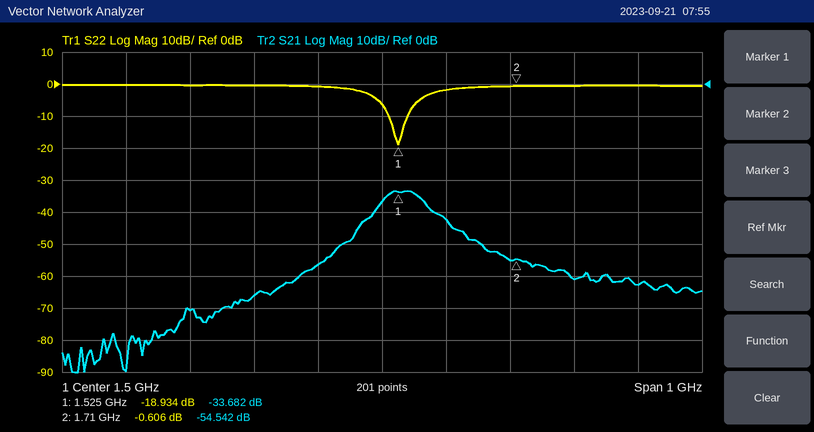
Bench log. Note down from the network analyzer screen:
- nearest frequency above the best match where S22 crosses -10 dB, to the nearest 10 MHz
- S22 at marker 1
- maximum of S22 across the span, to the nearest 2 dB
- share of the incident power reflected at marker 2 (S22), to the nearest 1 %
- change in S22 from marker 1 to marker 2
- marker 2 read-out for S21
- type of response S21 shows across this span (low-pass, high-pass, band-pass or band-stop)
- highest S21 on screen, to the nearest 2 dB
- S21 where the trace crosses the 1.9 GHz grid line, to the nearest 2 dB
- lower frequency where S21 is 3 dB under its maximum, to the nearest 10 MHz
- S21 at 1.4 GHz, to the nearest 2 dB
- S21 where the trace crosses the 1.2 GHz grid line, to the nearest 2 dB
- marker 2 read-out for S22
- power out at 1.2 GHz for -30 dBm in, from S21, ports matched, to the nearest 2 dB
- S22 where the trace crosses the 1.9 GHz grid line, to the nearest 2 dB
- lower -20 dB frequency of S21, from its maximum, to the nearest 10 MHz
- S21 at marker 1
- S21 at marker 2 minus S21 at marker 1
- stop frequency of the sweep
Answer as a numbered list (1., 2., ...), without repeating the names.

1. 1.54 GHz
2. -18.934 dB
3. 0 dB
4. 87 %
5. 18.328 dB
6. -54.542 dB
7. band-pass
8. -34 dB
9. -62 dB
10. 1.50 GHz
11. -56 dB
12. -70 dB
13. -0.606 dB
14. -100 dBm
15. 0 dB
16. 1.42 GHz
17. -33.682 dB
18. -20.860 dB
19. 2 GHz
